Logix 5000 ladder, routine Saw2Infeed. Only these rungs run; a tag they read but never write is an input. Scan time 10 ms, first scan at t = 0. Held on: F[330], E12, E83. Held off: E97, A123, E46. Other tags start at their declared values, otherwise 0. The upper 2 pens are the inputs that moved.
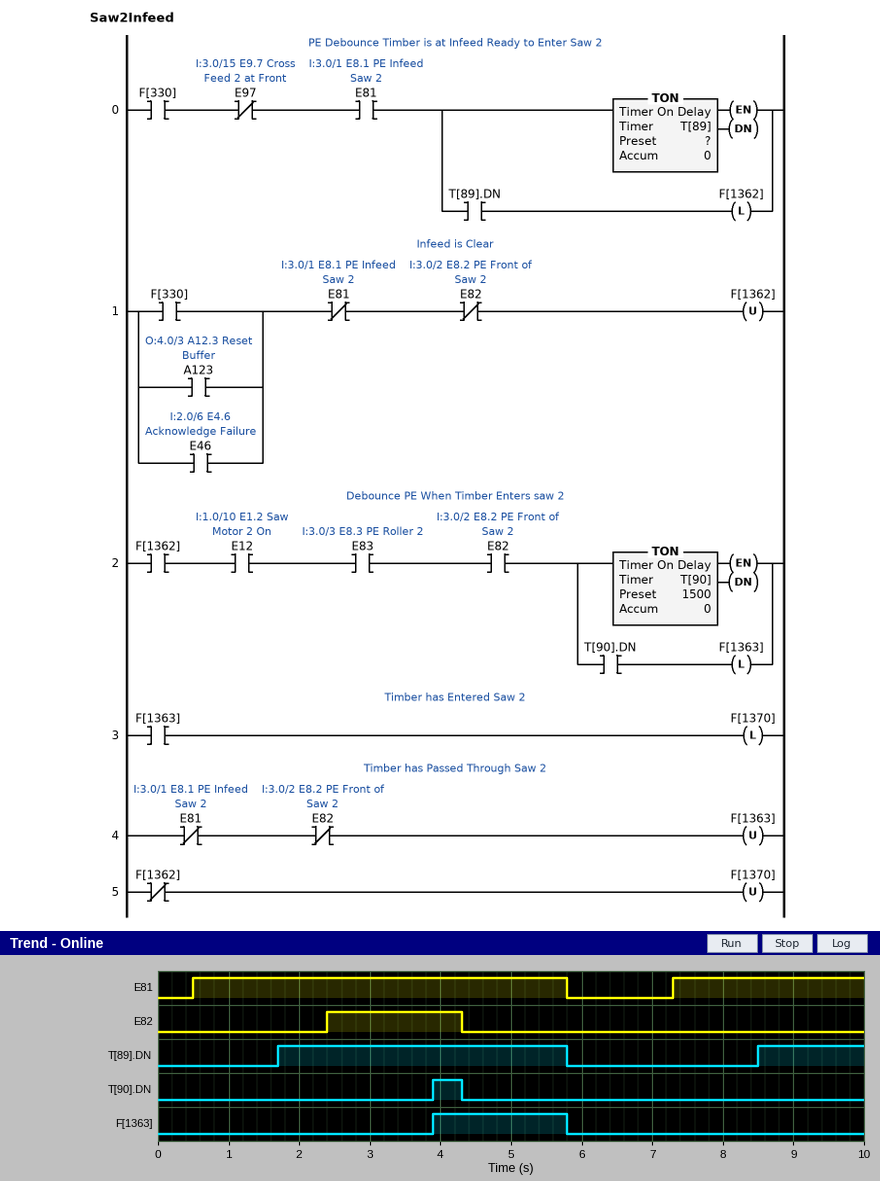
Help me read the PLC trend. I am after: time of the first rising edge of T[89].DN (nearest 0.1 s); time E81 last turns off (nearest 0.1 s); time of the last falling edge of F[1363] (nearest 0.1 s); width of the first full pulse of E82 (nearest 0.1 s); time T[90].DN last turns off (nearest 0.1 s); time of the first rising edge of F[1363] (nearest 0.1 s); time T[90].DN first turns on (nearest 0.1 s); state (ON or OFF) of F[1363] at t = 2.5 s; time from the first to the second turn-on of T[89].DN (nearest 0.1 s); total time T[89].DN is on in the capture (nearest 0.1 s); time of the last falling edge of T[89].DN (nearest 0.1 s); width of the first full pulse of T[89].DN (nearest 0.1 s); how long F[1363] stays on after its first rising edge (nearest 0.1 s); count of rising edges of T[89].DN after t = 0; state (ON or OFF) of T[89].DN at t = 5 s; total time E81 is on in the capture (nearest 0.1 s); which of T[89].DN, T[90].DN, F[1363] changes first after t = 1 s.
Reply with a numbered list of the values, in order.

1. 1.7 s
2. 5.8 s
3. 5.8 s
4. 1.9 s
5. 4.3 s
6. 3.9 s
7. 3.9 s
8. OFF
9. 6.8 s
10. 5.6 s
11. 5.8 s
12. 4.1 s
13. 1.9 s
14. 2
15. ON
16. 8.0 s
17. T[89].DN
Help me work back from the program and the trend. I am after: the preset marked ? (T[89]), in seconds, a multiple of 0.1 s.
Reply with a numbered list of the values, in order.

1. 1.2 s
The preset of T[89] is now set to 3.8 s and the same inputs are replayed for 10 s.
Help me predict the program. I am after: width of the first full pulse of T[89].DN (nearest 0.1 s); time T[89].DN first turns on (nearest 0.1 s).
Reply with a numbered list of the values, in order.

1. 1.5 s
2. 4.3 s
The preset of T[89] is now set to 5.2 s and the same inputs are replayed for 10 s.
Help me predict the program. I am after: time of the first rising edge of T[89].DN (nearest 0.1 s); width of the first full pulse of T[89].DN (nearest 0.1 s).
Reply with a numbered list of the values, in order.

1. 5.7 s
2. 0.1 s
